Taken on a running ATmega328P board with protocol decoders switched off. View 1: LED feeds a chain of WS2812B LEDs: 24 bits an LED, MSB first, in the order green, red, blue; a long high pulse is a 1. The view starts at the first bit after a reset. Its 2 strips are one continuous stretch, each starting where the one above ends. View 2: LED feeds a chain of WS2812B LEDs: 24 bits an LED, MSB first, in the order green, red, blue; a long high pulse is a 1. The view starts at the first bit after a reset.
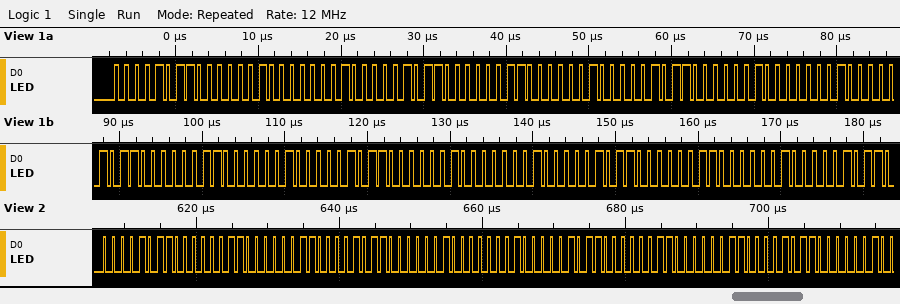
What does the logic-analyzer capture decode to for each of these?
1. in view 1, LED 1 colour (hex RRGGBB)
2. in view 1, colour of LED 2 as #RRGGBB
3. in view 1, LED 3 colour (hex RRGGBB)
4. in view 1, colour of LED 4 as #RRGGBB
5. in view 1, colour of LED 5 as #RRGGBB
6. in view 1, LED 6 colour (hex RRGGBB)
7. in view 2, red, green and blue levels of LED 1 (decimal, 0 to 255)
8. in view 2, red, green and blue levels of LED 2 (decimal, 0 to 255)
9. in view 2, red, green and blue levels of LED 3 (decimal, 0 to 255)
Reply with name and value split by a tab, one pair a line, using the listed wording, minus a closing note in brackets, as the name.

in view 1, LED 1 colour	#020B02
in view 1, colour of LED 2 as #RRGGBB	#030B02
in view 1, LED 3 colour	#020B02
in view 1, colour of LED 4 as #RRGGBB	#030B02
in view 1, colour of LED 5 as #RRGGBB	#020B02
in view 1, LED 6 colour	#030B02
in view 2, red, green and blue levels of LED 1	3, 11, 3
in view 2, red, green and blue levels of LED 2	2, 11, 2
in view 2, red, green and blue levels of LED 3	3, 11, 3
